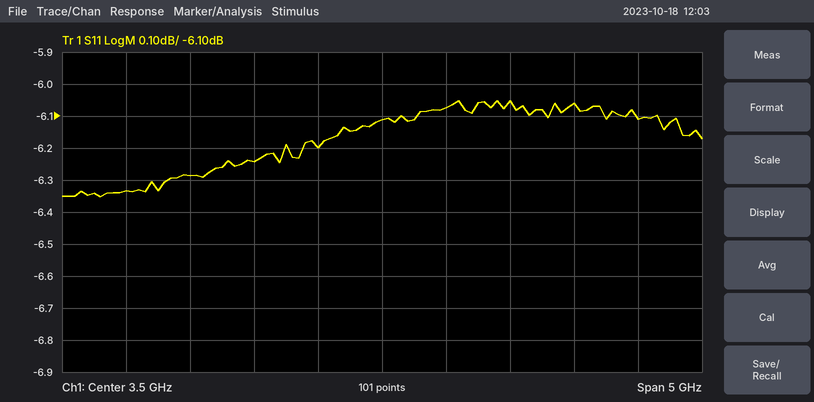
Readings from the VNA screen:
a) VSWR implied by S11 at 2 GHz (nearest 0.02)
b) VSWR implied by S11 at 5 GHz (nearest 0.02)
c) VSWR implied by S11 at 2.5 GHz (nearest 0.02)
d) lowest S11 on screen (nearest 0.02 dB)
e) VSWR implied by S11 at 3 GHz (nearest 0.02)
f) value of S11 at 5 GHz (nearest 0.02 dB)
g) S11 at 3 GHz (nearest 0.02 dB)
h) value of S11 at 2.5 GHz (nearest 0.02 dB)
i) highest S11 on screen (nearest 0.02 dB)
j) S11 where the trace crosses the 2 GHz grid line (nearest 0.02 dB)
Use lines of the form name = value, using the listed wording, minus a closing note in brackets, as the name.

VSWR implied by S11 at 2 GHz = 2.88
VSWR implied by S11 at 5 GHz = 2.98
VSWR implied by S11 at 2.5 GHz = 2.90
lowest S11 on screen = -6.36 dB
VSWR implied by S11 at 3 GHz = 2.92
value of S11 at 5 GHz = -6.06 dB
S11 at 3 GHz = -6.20 dB
value of S11 at 2.5 GHz = -6.24 dB
highest S11 on screen = -6.06 dB
S11 where the trace crosses the 2 GHz grid line = -6.28 dB
